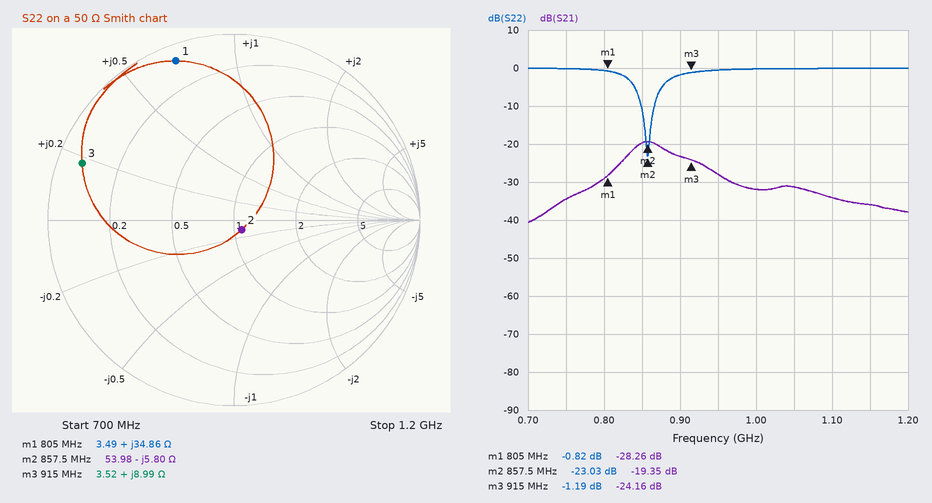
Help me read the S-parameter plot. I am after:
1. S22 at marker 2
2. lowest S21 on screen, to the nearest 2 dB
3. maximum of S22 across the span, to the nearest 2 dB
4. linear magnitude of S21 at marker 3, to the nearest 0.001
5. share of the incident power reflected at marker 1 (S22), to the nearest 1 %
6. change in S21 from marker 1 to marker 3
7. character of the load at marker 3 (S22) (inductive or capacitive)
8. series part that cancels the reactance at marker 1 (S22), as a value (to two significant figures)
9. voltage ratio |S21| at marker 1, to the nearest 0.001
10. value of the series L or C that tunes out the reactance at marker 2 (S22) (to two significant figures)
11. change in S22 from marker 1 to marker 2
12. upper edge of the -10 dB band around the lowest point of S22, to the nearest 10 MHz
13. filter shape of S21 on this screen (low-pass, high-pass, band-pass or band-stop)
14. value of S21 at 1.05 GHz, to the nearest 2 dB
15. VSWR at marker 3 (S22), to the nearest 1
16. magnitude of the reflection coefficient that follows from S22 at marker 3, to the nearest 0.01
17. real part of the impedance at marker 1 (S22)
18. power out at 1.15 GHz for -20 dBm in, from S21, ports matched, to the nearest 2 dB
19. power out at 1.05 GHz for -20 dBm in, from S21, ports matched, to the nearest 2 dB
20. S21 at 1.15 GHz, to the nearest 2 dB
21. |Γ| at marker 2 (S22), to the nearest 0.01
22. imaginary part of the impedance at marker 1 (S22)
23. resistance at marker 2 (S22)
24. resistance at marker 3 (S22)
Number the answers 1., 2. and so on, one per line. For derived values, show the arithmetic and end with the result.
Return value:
1. -23.03 dB
2. -40 dB
3. 0 dB
4. 10^(-24.16/20) ≈ 0.062
5. 10^(-0.82/10) ≈ 83 %
6. -24.16 − (-28.26) = 4.10 dB
7. inductive
8. C = 1/(2π × 805 MHz × 34.86 Ω) ≈ 5.7 pF
9. 10^(-28.26/20) ≈ 0.039
10. L = 5.8 Ω/(2π × 857.5 MHz) ≈ 1.1 nH
11. -23.03 − (-0.82) = -22.21 dB
12. 870 MHz
13. band-pass
14. -32 dB
15. 15
16. 10^(-1.19/20) ≈ 0.87
17. 3.49 Ω
18. -20 dBm + (-36 dB) = -56 dBm
19. -20 dBm + (-32 dB) = -52 dBm
20. -36 dB
21. 0.07
22. +34.86 Ω
23. 53.98 Ω
24. 3.52 Ω
